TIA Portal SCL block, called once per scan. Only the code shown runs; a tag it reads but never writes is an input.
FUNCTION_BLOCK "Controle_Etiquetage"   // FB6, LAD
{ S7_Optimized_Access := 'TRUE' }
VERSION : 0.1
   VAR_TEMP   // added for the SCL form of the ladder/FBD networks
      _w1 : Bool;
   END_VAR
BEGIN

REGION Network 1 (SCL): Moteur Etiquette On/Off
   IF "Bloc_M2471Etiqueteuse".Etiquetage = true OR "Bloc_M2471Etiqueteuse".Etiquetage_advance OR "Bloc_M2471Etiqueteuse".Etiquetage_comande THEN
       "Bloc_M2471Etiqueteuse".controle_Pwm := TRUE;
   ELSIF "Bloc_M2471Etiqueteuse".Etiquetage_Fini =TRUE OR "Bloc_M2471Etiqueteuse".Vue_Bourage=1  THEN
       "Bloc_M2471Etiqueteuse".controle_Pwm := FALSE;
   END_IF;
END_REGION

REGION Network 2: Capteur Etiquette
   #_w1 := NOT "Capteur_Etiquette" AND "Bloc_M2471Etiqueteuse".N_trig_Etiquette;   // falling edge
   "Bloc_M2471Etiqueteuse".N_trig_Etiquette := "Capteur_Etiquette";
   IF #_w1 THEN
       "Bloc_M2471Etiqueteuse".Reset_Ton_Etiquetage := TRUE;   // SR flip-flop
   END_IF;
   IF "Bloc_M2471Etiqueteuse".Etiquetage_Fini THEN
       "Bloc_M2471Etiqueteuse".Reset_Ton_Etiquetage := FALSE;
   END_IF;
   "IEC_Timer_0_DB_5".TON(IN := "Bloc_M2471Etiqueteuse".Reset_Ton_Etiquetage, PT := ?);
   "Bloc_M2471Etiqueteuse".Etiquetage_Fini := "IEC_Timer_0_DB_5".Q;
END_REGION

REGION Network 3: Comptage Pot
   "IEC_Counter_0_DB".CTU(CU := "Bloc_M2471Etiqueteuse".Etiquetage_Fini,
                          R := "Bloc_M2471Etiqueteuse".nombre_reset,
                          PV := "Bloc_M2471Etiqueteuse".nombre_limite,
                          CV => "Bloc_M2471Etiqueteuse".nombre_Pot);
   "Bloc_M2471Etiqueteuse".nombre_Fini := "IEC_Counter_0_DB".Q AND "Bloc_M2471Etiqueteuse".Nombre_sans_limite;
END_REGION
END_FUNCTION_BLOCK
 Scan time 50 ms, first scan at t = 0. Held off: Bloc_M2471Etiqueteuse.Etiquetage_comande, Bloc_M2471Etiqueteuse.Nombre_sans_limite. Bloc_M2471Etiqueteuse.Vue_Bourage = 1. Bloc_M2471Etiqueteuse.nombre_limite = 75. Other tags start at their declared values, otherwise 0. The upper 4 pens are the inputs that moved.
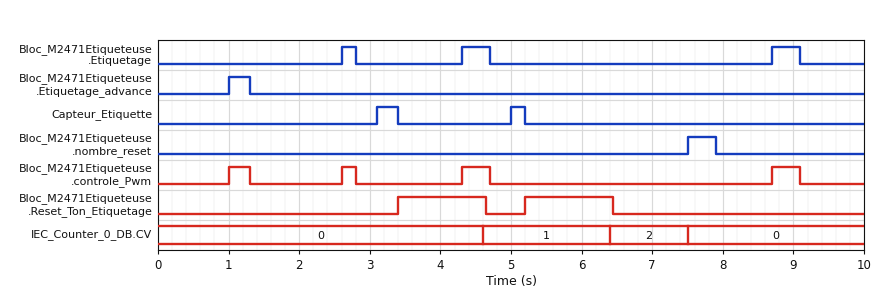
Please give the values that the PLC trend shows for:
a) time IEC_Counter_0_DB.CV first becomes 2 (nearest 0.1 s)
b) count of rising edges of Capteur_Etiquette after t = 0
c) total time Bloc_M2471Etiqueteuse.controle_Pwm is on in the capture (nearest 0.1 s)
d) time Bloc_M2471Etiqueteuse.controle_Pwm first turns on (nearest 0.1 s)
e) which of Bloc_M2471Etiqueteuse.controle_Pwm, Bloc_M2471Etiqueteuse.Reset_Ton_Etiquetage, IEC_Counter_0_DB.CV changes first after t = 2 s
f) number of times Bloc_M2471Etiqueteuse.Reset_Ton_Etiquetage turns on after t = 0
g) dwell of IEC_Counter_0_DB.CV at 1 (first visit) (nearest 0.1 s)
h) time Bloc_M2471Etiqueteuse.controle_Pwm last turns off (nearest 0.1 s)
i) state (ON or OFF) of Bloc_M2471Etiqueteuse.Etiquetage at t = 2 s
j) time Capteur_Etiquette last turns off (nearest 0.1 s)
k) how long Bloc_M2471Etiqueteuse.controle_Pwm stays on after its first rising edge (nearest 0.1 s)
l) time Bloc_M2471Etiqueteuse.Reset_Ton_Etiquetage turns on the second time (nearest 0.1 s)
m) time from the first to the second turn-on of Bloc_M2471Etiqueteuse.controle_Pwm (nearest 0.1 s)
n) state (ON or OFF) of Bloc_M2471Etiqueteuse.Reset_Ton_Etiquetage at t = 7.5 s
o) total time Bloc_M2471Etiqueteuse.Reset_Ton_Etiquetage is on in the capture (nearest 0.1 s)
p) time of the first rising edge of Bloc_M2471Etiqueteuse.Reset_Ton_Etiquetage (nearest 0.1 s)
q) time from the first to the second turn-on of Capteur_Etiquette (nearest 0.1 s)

6.4 s
2
1.3 s
1.0 s
Bloc_M2471Etiqueteuse.controle_Pwm
2
1.8 s
9.1 s
OFF
5.2 s
0.3 s
5.2 s
1.6 s
OFF
2.5 s
3.4 s
1.9 s
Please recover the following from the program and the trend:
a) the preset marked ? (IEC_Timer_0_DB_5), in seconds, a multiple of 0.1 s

1.2 s
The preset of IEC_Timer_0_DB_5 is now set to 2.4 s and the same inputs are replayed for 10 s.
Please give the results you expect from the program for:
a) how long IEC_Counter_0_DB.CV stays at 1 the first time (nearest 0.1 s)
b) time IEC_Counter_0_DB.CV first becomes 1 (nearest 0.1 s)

1.7 s
5.8 s
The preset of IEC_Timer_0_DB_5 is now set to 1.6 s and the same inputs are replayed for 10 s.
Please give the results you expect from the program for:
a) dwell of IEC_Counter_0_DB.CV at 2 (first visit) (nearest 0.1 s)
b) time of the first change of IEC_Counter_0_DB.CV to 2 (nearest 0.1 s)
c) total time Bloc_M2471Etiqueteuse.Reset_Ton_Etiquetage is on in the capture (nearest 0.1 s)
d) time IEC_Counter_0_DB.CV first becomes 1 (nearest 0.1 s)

0.7 s
6.8 s
3.3 s
5.0 s
